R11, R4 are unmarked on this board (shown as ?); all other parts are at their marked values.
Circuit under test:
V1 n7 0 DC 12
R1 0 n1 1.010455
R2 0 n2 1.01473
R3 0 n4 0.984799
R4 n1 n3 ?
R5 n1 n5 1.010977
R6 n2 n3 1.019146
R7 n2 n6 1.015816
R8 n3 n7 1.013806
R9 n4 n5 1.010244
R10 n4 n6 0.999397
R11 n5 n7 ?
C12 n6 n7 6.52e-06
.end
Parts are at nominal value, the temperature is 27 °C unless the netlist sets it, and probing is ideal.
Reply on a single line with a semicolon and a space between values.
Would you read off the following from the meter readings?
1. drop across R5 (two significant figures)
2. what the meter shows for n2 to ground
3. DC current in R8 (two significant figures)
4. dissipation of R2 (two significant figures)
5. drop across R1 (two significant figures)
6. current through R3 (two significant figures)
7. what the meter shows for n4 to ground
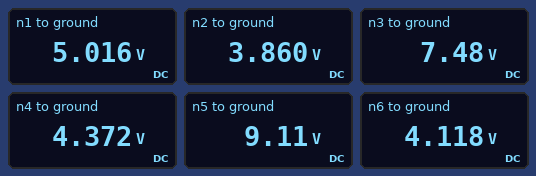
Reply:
4.1 V; 3.860 V; 4.5 A; 15 W; 5.0 V; 4.4 A; 4.372 V
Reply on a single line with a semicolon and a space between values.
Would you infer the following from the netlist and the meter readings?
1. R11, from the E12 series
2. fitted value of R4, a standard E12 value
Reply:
0.33 Ω; 2.7 Ω
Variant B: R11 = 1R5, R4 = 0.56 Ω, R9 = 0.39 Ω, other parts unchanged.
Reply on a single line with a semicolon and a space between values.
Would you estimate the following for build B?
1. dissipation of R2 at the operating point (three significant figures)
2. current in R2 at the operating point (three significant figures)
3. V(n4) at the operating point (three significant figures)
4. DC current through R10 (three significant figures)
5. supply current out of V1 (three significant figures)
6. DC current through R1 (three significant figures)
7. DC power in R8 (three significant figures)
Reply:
9.26 W; 3.02 A; 3.52 V; 225 mA; 10.7 A; 4.08 A; 36.5 W
